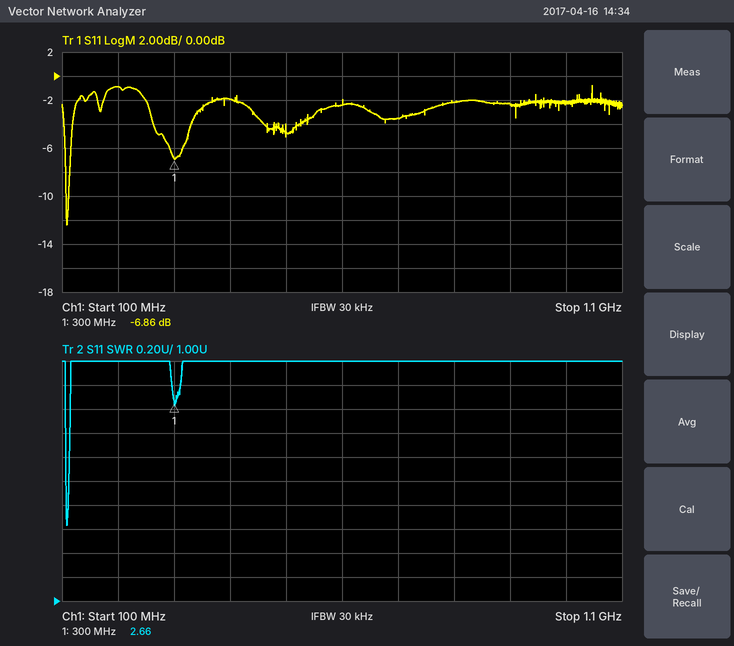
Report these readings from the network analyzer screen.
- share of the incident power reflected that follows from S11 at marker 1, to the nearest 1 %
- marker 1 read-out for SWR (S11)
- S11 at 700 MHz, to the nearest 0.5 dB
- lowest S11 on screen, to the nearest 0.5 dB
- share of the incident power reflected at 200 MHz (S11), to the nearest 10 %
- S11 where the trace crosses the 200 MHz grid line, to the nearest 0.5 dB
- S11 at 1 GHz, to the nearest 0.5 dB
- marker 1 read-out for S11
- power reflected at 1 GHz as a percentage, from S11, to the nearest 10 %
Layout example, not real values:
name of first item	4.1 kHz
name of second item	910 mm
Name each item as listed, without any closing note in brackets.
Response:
share of the incident power reflected that follows from S11 at marker 1, to the nearest 1 %	21 %
marker 1 read-out for SWR	2.66
S11 at 700 MHz, to the nearest 0.5 dB	-3.5 dB
lowest S11 on screen, to the nearest 0.5 dB	-12.5 dB
share of the incident power reflected at 200 MHz (S11), to the nearest 10 %	80 %
S11 where the trace crosses the 200 MHz grid line, to the nearest 0.5 dB	-1.0 dB
S11 at 1 GHz, to the nearest 0.5 dB	-2.0 dB
marker 1 read-out for S11	-6.86 dB
power reflected at 1 GHz as a percentage, from S11, to the nearest 10 %	60 %
